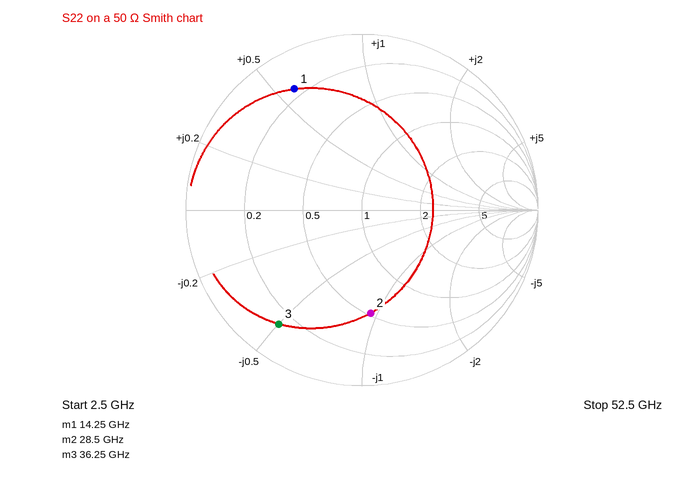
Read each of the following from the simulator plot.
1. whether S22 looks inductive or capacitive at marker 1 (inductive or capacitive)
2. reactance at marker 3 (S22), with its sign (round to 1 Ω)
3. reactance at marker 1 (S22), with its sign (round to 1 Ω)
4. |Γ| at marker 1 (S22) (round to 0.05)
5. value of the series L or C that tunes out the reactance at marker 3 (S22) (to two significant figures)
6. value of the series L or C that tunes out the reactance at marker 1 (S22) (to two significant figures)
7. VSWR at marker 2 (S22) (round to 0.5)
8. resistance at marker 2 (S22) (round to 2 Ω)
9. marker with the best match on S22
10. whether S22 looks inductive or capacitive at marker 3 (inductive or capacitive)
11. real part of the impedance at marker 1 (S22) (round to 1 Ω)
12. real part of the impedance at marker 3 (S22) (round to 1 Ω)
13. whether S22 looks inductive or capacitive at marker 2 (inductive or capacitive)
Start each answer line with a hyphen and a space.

- inductive
- -25 Ω
- +29 Ω
- 0.80
- 110 pH
- 390 fF
- 4.0
- 26 Ω
- marker 2
- capacitive
- 8 Ω
- 7 Ω
- capacitive
